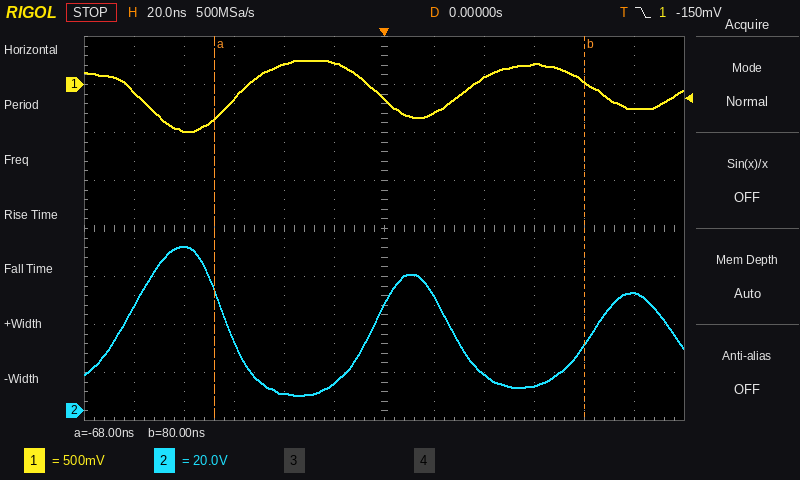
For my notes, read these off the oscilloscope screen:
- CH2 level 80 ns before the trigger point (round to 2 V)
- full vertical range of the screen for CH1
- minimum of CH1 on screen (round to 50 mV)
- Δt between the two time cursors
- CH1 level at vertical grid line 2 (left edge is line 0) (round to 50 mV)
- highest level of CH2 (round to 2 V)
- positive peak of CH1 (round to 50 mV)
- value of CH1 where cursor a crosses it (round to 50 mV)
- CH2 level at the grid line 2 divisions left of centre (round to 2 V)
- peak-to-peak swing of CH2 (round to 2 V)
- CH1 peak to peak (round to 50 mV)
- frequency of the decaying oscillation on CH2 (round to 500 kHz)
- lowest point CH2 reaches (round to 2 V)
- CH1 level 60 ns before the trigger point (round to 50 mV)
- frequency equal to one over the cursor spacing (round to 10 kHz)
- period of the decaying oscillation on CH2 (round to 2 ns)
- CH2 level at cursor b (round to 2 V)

68 V
4 V
-500 mV
148 ns
-500 mV
68 V
250 mV
-350 mV
8 V
62 V
750 mV
11.0 MHz
6 V
-150 mV
6.76 MHz
90 ns
28 V
